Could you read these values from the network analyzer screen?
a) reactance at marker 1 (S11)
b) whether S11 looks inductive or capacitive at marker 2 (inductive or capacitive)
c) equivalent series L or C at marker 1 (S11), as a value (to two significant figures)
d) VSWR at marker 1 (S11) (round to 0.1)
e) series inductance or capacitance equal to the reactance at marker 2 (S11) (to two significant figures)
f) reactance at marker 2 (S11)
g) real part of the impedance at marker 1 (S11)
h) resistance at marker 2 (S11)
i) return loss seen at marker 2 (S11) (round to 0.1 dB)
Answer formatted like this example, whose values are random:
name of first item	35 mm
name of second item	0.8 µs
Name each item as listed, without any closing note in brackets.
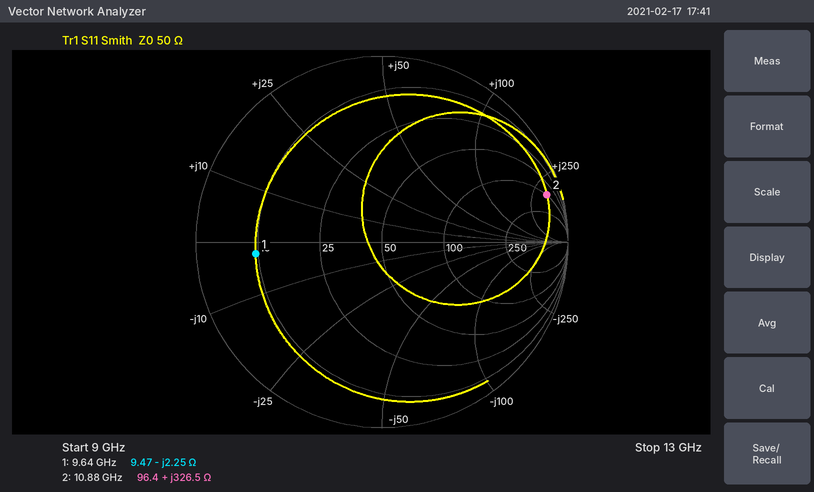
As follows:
reactance at marker 1	-2.25 Ω
whether S11 looks inductive or capacitive at marker 2	inductive
equivalent series L or C at marker 1 (S11), as a value	7.3 pF
VSWR at marker 1 (S11)	5.3
series inductance or capacitance equal to the reactance at marker 2 (S11)	4.8 nH
reactance at marker 2	+326.5 Ω
real part of the impedance at marker 1	9.47 Ω
resistance at marker 2	96.4 Ω
return loss seen at marker 2 (S11)	0.7 dB
